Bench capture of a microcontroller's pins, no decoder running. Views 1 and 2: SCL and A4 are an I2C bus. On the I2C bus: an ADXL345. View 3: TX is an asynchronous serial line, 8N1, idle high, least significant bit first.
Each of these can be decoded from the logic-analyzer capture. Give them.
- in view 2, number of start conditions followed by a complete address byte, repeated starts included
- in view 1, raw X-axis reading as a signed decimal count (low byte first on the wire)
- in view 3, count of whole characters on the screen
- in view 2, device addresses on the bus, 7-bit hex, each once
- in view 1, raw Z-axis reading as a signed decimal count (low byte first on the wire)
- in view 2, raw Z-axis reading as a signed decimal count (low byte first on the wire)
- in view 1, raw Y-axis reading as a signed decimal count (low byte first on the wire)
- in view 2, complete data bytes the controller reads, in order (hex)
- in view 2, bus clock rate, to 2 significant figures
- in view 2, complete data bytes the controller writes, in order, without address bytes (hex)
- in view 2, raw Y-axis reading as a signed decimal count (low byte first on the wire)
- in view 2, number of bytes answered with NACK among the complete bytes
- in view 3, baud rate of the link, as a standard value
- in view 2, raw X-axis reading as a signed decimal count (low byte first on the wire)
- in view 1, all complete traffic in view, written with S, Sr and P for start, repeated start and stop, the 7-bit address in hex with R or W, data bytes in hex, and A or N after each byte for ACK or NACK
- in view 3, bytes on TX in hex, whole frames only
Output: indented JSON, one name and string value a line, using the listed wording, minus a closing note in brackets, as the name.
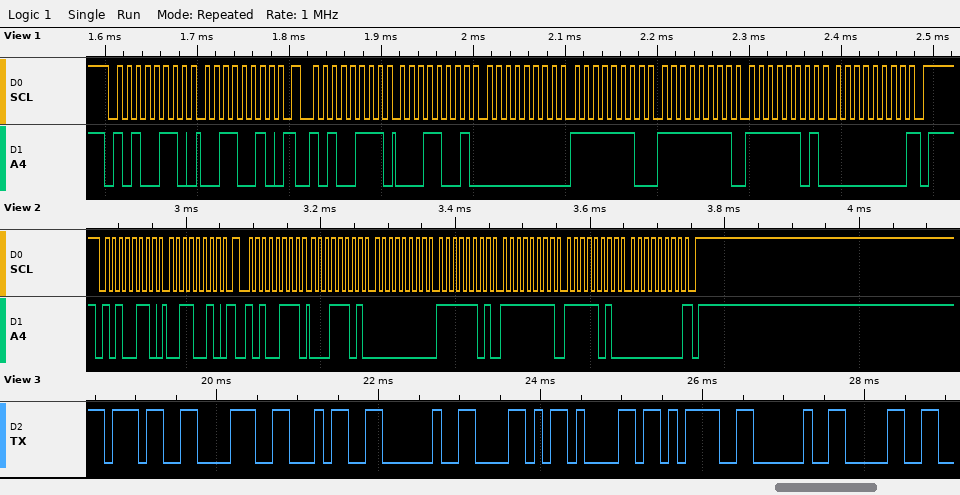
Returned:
{
  "in view 2, number of start conditions followed by a complete address byte, repeated starts included": "2",
  "in view 1, raw X-axis reading as a signed decimal count": "25",
  "in view 3, count of whole characters on the screen": "9",
  "in view 2, device addresses on the bus, 7-bit hex, each once": "0x53",
  "in view 1, raw Z-axis reading as a signed decimal count": "253",
  "in view 2, raw Z-axis reading as a signed decimal count": "250",
  "in view 1, raw Y-axis reading as a signed decimal count": "-2",
  "in view 2, complete data bytes the controller reads, in order": "1D 00 FD FF FA 00",
  "in view 2, bus clock rate, to 2 significant figures": "100 kHz",
  "in view 2, complete data bytes the controller writes, in order, without address bytes": "32",
  "in view 2, raw Y-axis reading as a signed decimal count": "-3",
  "in view 2, number of bytes answered with NACK among the complete bytes": "1",
  "in view 3, baud rate of the link, as a standard value": "9600 baud",
  "in view 2, raw X-axis reading as a signed decimal count": "29",
  "in view 1, all complete traffic in view, written with S, Sr and P for start, repeated start and stop, the 7-bit address in hex with R or W, data bytes in hex, and A or N after each byte for ACK or NACK": "S 53W A 32 A Sr 53R A 19 A 00 A FE A FF A FD A 00 N P",
  "in view 3, bytes on TX in hex, whole frames only": "37 38 34 20 58 61 3D 20 30"
}
